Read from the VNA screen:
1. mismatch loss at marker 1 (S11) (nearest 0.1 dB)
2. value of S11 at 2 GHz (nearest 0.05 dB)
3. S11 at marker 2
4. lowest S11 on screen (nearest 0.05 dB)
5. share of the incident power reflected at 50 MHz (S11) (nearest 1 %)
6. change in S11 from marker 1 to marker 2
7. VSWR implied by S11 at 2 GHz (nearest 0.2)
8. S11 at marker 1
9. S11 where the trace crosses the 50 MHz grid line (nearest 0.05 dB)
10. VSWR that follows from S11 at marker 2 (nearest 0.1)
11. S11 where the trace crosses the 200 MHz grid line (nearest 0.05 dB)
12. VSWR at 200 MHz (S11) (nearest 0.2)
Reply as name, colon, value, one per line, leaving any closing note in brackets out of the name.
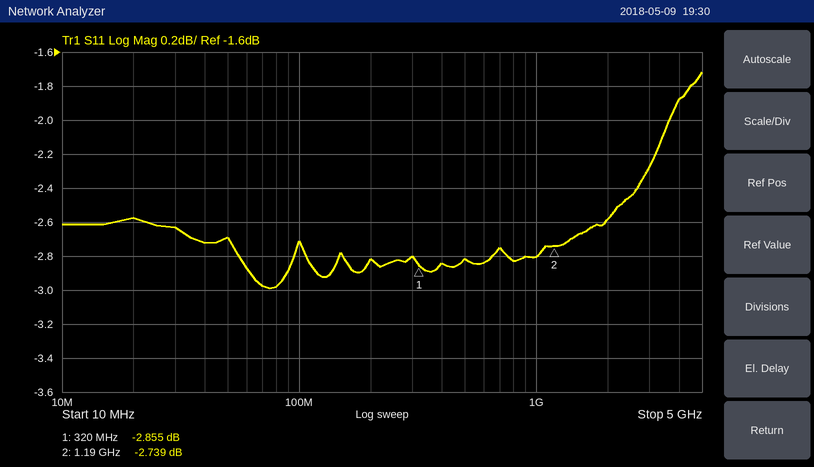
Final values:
mismatch loss at marker 1 (S11): 3.2 dB
value of S11 at 2 GHz: -2.60 dB
S11 at marker 2: -2.739 dB
lowest S11 on screen: -3.00 dB
share of the incident power reflected at 50 MHz (S11): 54 %
change in S11 from marker 1 to marker 2: 0.116 dB
VSWR implied by S11 at 2 GHz: 6.8
S11 at marker 1: -2.855 dB
S11 where the trace crosses the 50 MHz grid line: -2.70 dB
VSWR that follows from S11 at marker 2: 6.4
S11 where the trace crosses the 200 MHz grid line: -2.80 dB
VSWR at 200 MHz (S11): 6.2
